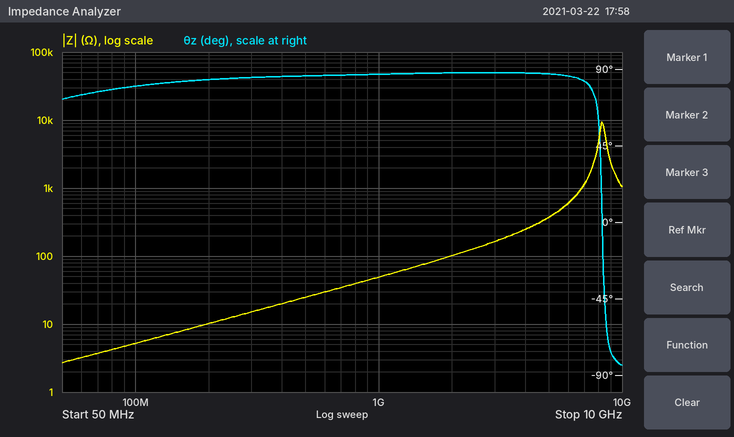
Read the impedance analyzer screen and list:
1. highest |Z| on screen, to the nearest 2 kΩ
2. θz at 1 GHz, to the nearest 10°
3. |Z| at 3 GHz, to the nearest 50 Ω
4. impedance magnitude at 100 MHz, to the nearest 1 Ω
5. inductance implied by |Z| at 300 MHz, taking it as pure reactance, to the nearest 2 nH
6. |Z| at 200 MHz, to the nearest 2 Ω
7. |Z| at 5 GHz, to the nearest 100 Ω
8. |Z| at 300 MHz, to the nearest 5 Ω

10 kΩ
90°
150 Ω
5 Ω
8 nH
10 Ω
400 Ω
15 Ω
